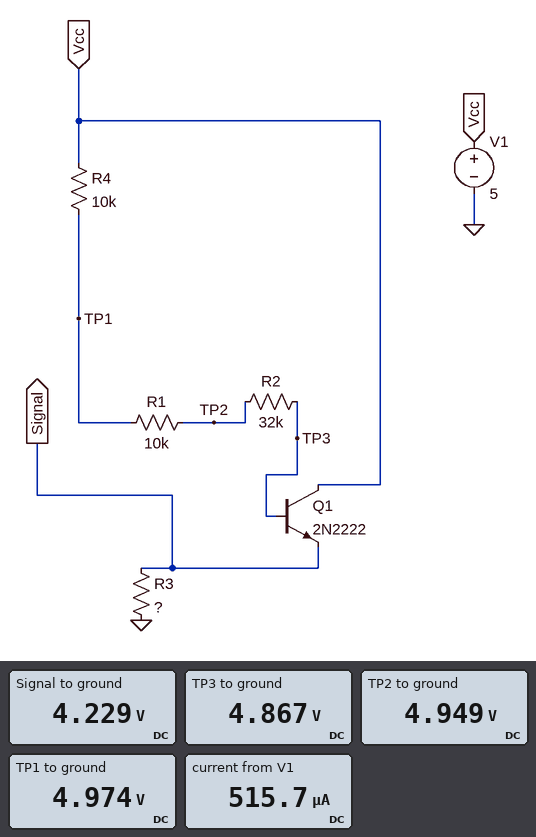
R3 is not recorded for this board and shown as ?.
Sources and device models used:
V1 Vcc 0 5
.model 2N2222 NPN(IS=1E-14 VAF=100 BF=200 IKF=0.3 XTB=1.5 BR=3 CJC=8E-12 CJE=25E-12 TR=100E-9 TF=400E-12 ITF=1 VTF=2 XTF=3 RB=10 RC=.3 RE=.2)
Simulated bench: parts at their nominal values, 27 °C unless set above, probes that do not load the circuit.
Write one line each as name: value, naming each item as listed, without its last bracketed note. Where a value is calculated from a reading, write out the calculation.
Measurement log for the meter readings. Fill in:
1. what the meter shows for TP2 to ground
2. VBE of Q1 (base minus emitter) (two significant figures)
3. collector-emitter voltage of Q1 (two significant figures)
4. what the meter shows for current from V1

what the meter shows for TP2 to ground: 4.949 V
VBE of Q1 (base minus emitter): 4.867 V - 4.229 V = 640 mV
collector-emitter voltage of Q1: 5 V - 4.229 V = 770 mV
what the meter shows for current from V1: 515.7 µA
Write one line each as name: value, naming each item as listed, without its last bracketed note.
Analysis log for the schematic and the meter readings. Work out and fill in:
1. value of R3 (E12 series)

value of R3: 8.2 kΩ
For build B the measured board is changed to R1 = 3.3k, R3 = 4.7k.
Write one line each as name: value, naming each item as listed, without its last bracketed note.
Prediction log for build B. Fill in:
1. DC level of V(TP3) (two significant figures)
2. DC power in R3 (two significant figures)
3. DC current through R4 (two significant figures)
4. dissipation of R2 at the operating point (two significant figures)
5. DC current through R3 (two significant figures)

DC level of V(TP3): 4.8 V
DC power in R3: 3.7 mW
DC current through R4: 4.4 µA
dissipation of R2 at the operating point: 620 nW
DC current through R3: 880 µA
